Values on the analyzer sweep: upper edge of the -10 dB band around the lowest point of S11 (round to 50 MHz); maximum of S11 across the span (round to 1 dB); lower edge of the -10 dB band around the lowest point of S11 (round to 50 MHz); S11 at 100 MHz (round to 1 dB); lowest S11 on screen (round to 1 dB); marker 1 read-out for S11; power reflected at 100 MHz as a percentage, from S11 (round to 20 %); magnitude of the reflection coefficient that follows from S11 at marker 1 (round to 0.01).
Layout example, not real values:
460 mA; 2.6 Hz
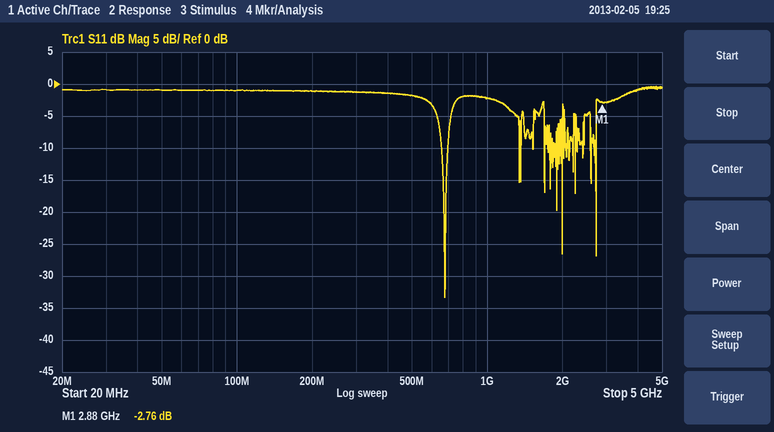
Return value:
700 MHz; 0 dB; 650 MHz; -1 dB; -33 dB; -2.76 dB; 80 %; 0.73
